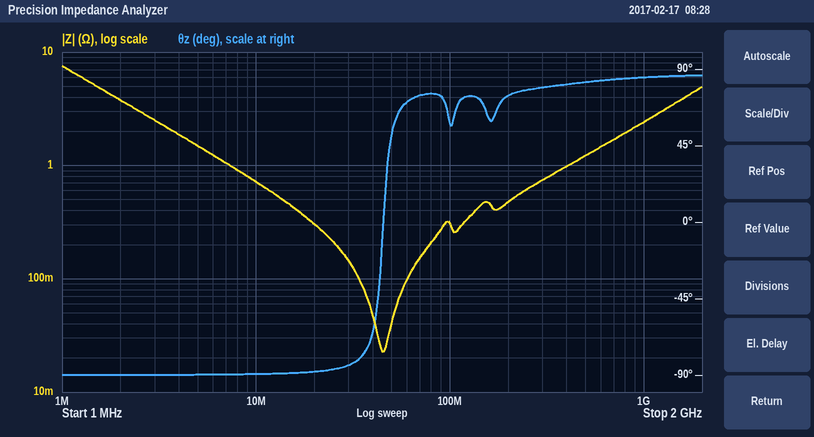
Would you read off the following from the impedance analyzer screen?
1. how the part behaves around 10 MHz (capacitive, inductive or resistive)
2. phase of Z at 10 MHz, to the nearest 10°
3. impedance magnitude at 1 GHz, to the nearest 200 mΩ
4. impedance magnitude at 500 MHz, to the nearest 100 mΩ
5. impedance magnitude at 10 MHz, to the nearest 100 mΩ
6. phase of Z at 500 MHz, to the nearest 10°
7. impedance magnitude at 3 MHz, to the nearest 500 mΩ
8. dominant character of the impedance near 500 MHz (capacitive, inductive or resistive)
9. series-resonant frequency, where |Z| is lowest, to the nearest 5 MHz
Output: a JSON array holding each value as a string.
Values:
["capacitive", "-90°", "2.4 Ω", "1.2 Ω", "700 mΩ", "80°", "2.5 Ω", "inductive", "45 MHz"]
